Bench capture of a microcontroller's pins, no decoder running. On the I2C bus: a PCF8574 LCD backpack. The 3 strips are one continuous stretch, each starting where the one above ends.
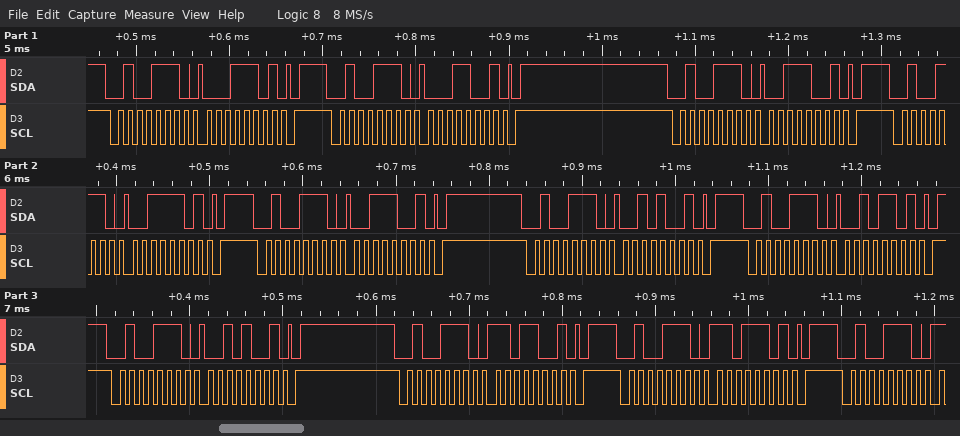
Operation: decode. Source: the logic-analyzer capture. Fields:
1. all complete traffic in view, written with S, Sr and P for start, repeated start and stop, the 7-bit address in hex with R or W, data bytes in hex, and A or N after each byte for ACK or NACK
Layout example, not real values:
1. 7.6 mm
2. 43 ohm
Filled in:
1. S 27W A 1D A P S 27W A 19 A P S 27W A 39 A P S 27W A 3D A P S 27W A 39 A P S 27W A 29 A P S 27W A 2D A P S 27W A 29 A P S 27W A D9 A P S 27W A DD A P S 27W A
